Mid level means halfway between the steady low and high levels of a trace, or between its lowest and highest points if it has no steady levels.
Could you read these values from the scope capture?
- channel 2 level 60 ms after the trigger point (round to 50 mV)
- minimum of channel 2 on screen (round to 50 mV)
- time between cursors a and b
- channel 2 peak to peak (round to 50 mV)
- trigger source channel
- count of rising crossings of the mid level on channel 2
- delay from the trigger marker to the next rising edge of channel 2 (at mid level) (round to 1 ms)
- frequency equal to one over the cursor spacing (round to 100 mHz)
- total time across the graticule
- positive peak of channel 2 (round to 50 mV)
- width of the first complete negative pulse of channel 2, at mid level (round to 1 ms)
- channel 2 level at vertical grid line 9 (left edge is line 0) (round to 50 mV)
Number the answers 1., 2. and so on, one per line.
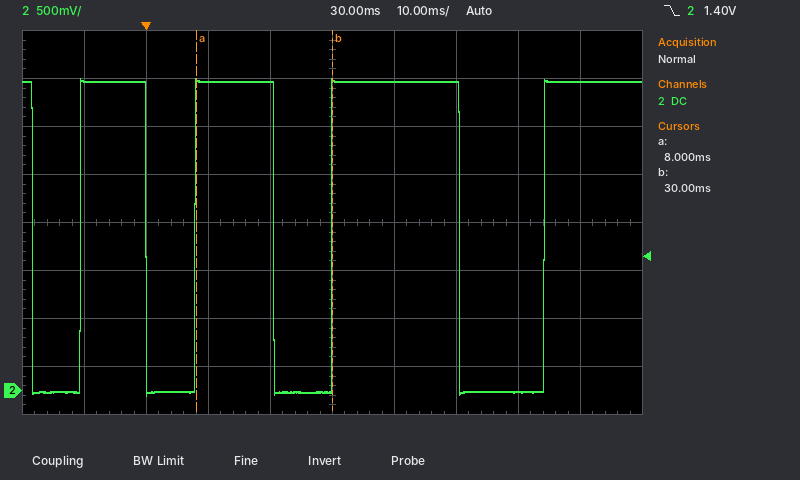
1. 0 mV
2. -50 mV
3. 22 ms
4. 3.30 V
5. channel 2
6. 4
7. 8 ms
8. 45.5 Hz
9. 100 ms
10. 3.25 V
11. 8 ms
12. 3.20 V
